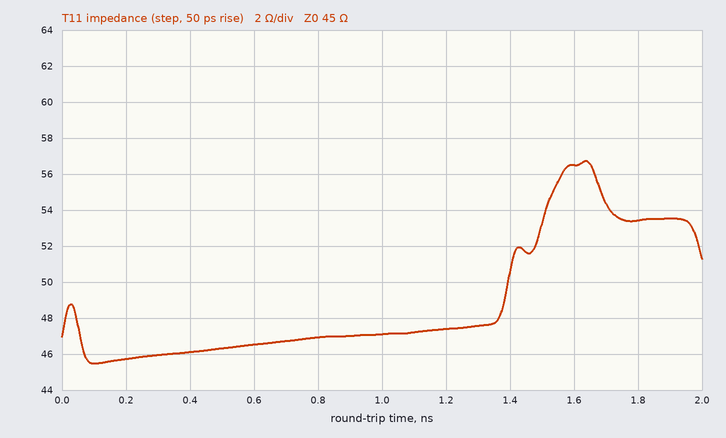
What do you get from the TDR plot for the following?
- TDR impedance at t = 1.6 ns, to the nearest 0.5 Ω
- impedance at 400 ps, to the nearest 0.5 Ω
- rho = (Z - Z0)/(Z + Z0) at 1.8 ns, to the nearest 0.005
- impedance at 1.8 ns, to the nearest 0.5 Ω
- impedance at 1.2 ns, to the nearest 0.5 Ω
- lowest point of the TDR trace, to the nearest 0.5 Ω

56.5 Ω
46.0 Ω
+0.085
53.5 Ω
47.5 Ω
45.5 Ω
